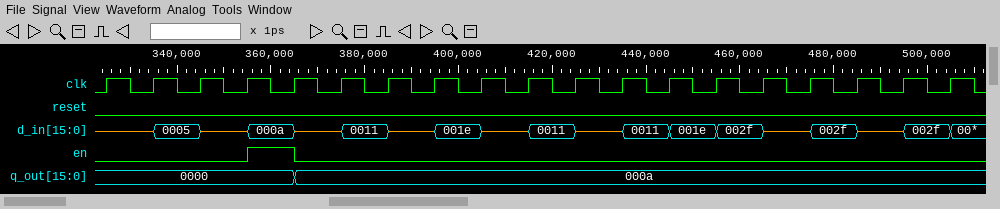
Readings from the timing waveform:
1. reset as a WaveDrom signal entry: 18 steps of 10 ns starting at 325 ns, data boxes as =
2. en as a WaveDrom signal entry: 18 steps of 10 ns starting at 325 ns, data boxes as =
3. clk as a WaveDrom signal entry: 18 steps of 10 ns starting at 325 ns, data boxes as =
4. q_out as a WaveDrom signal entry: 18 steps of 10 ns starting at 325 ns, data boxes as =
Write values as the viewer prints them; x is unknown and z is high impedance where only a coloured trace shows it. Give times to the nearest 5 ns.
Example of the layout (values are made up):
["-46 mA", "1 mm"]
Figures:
["{name: 'reset', wave: '0.................'}", "{name: 'en', wave: '0..10.............'}", "{name: 'clk', wave: 'p.................'}", "{name: 'q_out', wave: '=...=.............', data: '0000 000a'}"]
